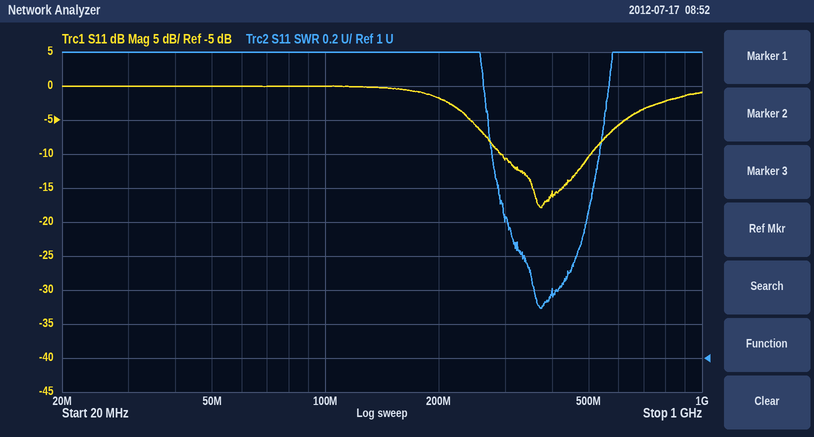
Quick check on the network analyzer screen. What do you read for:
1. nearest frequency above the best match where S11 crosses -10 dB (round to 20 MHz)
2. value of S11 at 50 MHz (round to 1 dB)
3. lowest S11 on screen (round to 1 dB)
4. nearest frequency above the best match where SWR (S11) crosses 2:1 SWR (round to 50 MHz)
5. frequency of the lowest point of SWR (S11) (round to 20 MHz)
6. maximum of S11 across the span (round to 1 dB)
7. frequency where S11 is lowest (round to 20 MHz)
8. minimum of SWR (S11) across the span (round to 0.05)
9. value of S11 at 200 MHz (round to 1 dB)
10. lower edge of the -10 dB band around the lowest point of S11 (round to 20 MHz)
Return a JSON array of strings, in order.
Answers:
["500 MHz", "0 dB", "-18 dB", "500 MHz", "380 MHz", "0 dB", "380 MHz", "1.30", "-2 dB", "300 MHz"]
